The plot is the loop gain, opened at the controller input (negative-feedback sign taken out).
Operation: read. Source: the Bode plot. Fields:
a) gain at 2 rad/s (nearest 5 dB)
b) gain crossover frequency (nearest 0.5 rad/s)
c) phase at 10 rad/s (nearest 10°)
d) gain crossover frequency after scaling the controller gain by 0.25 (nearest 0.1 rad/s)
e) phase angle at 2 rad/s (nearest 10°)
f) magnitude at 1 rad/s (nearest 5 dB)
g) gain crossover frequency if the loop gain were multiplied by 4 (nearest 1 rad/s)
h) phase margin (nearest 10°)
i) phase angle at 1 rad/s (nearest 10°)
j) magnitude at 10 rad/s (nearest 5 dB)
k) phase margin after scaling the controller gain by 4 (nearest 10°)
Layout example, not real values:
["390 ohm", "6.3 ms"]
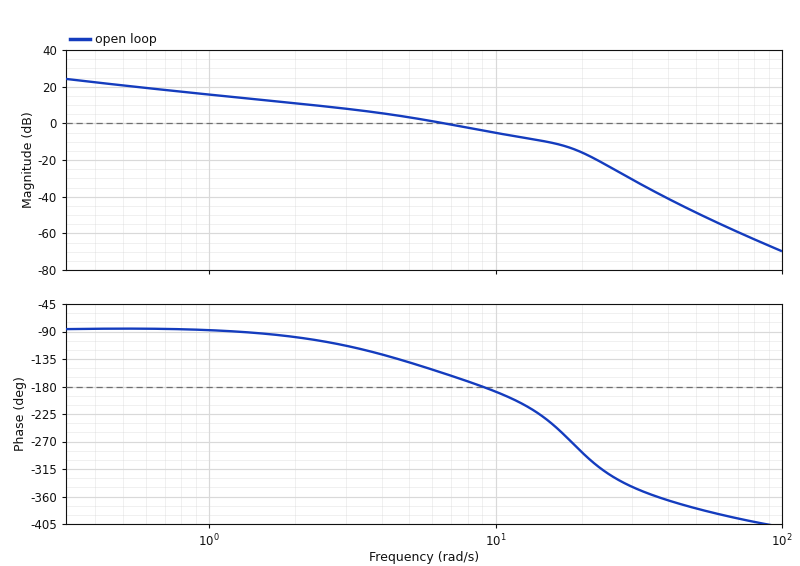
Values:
["10 dB", "6.5 rad/s", "-190°", "1.7 rad/s", "-100°", "15 dB", "17 rad/s", "20°", "-90°", "-5 dB", "-80°"]
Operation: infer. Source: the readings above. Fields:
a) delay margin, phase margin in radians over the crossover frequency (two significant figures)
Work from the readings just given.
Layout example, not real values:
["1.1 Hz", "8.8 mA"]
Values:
["0.054 s"]
